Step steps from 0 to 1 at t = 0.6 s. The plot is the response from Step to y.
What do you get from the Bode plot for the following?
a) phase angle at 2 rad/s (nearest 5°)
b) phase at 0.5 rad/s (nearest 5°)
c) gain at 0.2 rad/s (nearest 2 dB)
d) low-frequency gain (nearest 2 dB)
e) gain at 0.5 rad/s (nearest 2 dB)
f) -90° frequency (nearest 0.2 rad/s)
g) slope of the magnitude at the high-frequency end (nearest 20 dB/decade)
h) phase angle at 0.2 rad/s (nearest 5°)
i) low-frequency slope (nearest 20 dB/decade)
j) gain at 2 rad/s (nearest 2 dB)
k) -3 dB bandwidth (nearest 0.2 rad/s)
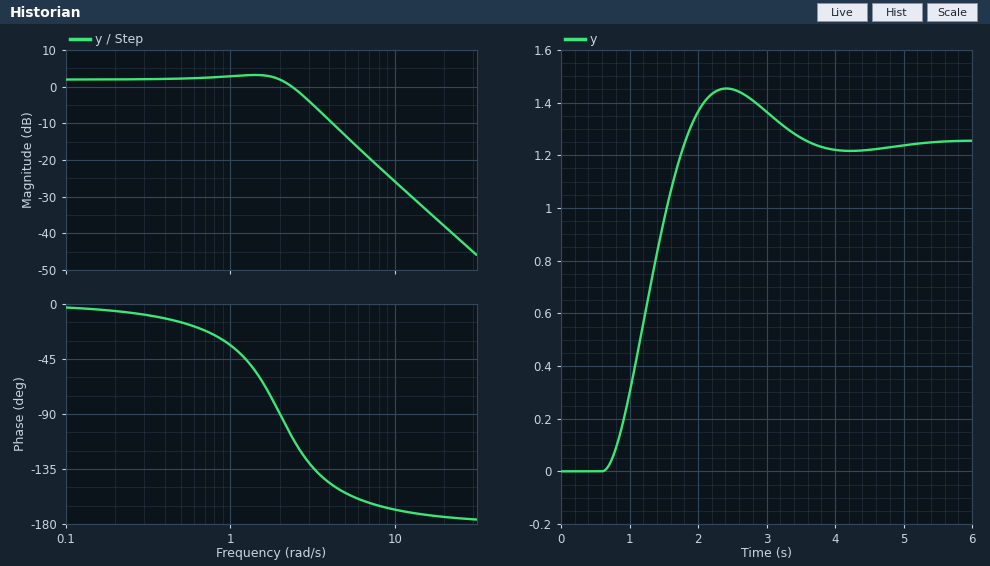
-90°
-15°
2 dB
2 dB
2 dB
2.0 rad/s
-40 dB/decade
-5°
0 dB/decade
2 dB
2.6 rad/s
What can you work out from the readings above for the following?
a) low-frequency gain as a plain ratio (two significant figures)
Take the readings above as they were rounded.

1.3
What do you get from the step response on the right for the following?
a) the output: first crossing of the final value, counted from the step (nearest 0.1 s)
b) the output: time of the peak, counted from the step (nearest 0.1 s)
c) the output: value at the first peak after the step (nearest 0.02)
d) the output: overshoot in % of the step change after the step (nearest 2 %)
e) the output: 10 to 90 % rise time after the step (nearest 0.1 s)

1.2 s
1.8 s
1.46
16 %
0.8 s
